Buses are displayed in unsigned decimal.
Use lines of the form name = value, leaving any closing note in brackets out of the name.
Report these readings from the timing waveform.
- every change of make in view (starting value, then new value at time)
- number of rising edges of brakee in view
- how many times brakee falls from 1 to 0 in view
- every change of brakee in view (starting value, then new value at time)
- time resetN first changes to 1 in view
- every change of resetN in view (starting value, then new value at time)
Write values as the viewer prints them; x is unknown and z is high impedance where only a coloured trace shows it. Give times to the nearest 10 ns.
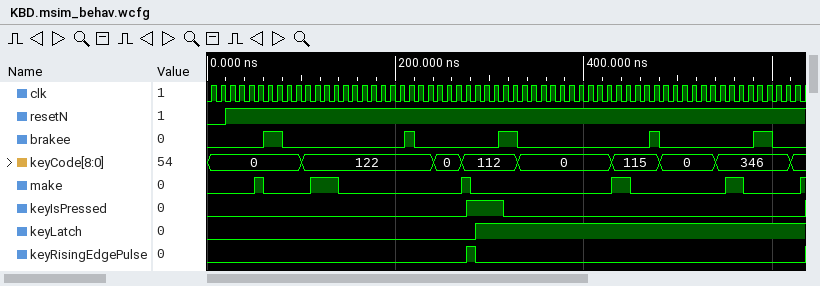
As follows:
every change of make in view = 0, 1 at 50 ns, 0 at 60 ns, 1 at 110 ns, 0 at 140 ns, 1 at 270 ns, 0 at 280 ns, 1 at 430 ns, 0 at 450 ns, 1 at 550 ns, 0 at 570 ns, 1 at 630 ns
number of rising edges of brakee in view = 5
how many times brakee falls from 1 to 0 in view = 5
every change of brakee in view = 0, 1 at 60 ns, 0 at 80 ns, 1 at 210 ns, 0 at 220 ns, 1 at 310 ns, 0 at 330 ns, 1 at 470 ns, 0 at 480 ns, 1 at 580 ns, 0 at 600 ns
time resetN first changes to 1 in view = 20 ns
every change of resetN in view = 0, 1 at 20 ns
